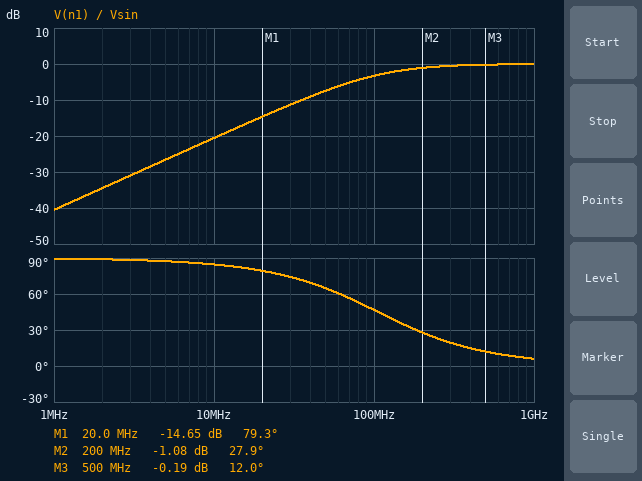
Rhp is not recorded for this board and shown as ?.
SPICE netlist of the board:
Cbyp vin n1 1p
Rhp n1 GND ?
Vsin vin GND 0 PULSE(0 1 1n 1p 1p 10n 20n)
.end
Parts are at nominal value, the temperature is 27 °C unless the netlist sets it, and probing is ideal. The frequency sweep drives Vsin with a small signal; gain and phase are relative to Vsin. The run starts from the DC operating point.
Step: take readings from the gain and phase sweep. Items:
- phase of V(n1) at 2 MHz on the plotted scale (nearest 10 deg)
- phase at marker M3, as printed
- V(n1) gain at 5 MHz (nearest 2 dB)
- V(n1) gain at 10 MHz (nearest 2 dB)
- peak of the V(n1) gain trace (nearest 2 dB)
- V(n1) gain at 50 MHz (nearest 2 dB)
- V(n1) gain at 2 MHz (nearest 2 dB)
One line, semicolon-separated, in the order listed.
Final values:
90 deg; 12.0 deg; -26 dB; -20 dB; 0 dB; -8 dB; -34 dB
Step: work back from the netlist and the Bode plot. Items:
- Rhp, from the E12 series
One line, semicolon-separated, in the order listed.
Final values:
1.5 kΩ
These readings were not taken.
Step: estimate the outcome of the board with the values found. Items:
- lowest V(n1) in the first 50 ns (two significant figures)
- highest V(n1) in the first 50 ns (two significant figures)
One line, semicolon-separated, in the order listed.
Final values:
-1.0 V; 1.0 V
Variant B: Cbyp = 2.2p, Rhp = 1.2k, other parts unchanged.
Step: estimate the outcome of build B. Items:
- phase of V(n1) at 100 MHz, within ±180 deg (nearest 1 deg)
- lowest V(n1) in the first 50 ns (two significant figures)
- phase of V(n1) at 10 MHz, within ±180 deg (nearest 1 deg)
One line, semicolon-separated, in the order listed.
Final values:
31 deg; -980 mV; 81 deg
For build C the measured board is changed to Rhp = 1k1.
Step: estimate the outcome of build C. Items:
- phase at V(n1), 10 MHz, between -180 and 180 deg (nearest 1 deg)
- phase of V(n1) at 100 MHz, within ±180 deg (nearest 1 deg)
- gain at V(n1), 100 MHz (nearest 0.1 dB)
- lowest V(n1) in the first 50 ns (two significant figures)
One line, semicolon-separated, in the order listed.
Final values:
86 deg; 55 deg; -4.9 dB; -1.0 V
